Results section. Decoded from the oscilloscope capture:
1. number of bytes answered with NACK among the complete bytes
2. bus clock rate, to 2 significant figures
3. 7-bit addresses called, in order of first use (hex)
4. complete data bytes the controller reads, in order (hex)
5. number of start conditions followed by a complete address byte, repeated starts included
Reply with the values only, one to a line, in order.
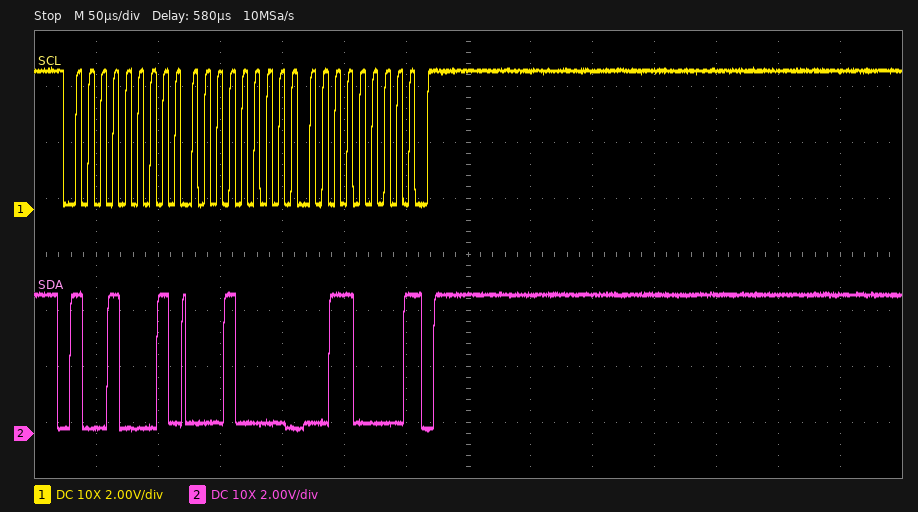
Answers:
1
100 kHz
0x48
10 30
1
